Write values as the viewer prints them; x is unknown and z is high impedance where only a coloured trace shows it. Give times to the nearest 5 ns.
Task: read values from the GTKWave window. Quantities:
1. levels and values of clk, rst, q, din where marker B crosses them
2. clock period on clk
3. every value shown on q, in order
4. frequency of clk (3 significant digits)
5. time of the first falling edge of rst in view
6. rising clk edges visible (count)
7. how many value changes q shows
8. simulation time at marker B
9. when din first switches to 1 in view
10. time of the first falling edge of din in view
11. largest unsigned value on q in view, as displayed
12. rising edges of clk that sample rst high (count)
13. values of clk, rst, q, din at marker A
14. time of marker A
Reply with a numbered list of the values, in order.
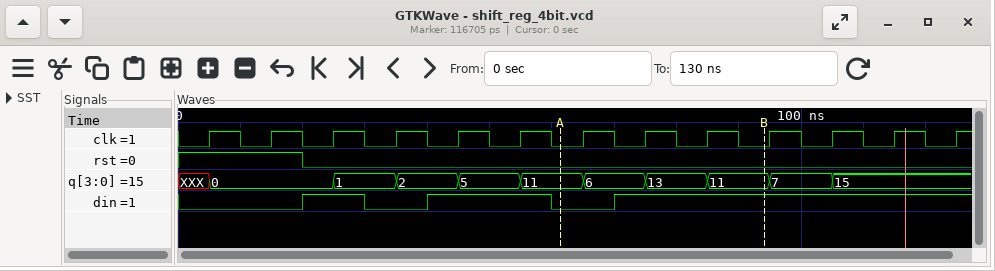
1. clk=0, rst=0, q=11, din=1
2. 10 ns
3. XXX, 0, 1, 2, 5, 11, 6, 13, 11, 7, 15
4. 100 MHz
5. 20 ns
6. 13
7. 10
8. 95 ns
9. 20 ns
10. 30 ns
11. 15
12. 2
13. clk=0, rst=0, q=11, din=0
14. 60 ns
